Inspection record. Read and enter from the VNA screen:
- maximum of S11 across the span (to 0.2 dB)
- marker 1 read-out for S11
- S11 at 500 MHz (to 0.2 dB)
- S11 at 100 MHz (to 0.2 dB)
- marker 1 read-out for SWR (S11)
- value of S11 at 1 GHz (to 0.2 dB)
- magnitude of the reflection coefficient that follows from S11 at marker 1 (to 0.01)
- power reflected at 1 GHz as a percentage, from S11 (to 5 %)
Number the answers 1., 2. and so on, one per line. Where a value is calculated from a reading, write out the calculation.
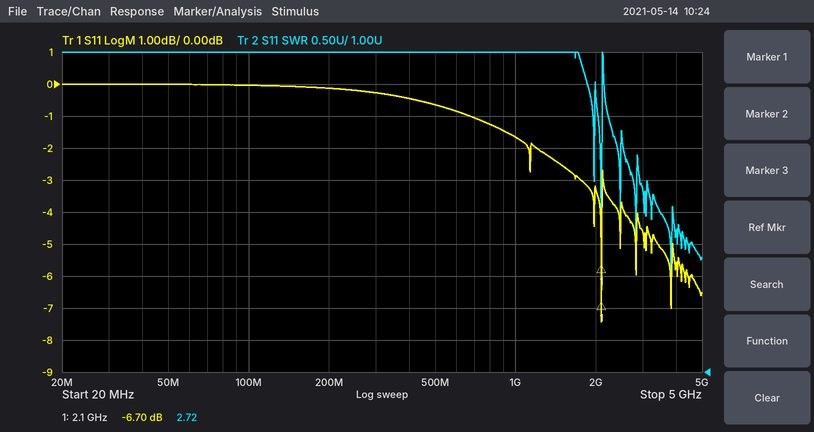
1. 0.0 dB
2. -6.70 dB
3. -0.6 dB
4. 0.0 dB
5. 2.72
6. -1.6 dB
7. 10^(-6.7/20) ≈ 0.46
8. 10^(-1.6/10) ≈ 69.2 %, so 70 % to the nearest 5 %
